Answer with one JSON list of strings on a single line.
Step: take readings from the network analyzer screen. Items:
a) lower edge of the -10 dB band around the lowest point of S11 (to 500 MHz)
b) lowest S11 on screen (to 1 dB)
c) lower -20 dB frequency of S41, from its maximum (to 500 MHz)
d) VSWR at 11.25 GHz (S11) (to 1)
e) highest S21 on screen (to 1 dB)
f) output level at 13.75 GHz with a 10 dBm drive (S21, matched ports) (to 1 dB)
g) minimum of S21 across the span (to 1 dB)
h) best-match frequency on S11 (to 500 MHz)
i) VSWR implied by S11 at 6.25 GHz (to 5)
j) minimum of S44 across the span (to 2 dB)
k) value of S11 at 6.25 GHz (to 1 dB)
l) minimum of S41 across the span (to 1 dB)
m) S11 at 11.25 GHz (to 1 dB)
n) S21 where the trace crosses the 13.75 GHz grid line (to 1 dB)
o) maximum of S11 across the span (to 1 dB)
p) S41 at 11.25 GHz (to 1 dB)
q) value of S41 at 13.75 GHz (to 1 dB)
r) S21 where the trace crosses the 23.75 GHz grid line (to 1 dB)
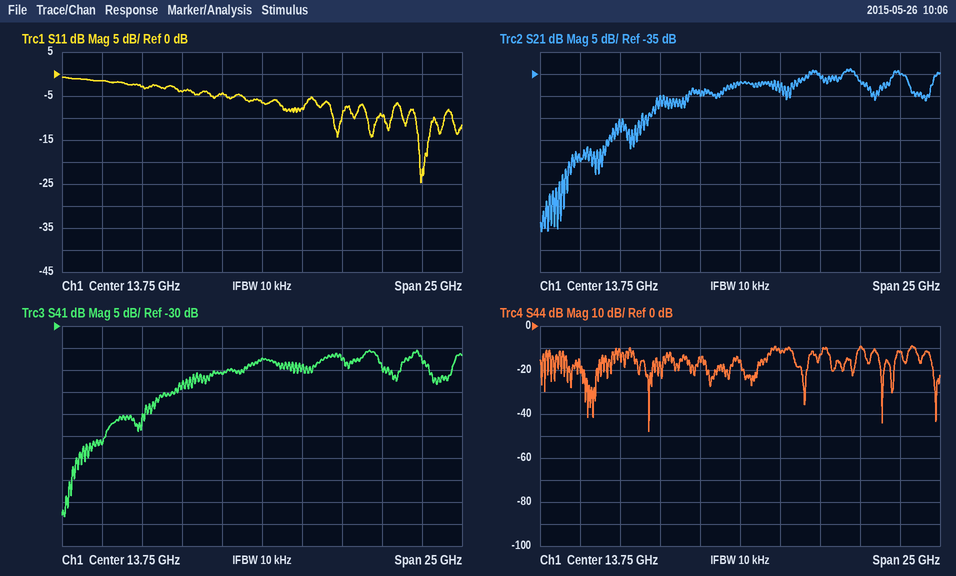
["23.5 GHz", "-25 dB", "4.0 GHz", "4", "-34 dB", "-27 dBm", "-71 dB", "23.5 GHz", "5", "-48 dB", "-3 dB", "-73 dB", "-4 dB", "-37 dB", "-1 dB", "-41 dB", "-37 dB", "-35 dB"]
